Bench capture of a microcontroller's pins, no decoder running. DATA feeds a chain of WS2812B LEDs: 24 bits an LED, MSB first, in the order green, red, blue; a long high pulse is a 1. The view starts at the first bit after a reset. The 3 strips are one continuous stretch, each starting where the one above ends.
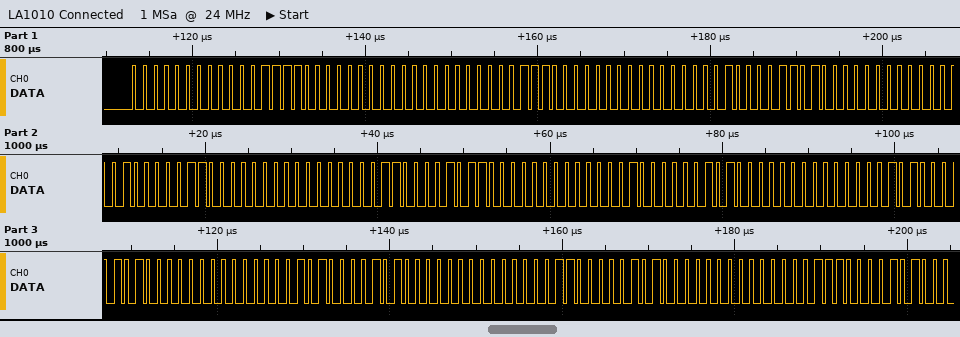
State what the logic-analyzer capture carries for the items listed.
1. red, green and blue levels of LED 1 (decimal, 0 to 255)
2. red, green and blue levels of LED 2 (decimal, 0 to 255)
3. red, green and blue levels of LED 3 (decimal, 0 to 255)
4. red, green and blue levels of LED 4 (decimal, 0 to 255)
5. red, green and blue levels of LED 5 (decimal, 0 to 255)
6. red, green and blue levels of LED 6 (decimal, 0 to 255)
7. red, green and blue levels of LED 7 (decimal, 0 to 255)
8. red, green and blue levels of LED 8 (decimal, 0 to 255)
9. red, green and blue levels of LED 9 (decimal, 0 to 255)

15, 0, 0
14, 0, 0
13, 1, 0
12, 2, 0
11, 3, 0
10, 4, 0
10, 5, 0
10, 5, 0
10, 6, 0
